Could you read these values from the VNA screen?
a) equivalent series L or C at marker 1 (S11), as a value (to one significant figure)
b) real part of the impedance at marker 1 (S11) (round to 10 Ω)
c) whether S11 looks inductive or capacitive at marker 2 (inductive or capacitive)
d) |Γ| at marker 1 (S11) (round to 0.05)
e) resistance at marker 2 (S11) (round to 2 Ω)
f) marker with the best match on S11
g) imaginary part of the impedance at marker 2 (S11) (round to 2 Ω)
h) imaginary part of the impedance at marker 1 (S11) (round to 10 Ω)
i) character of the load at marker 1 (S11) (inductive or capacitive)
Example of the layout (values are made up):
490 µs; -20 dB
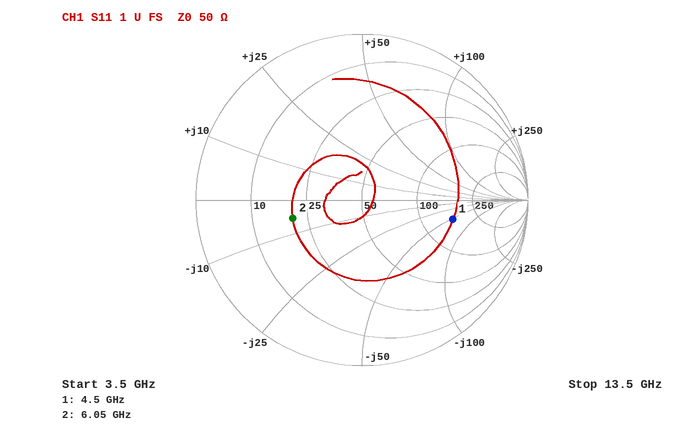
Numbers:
700 fF; 160 Ω; capacitive; 0.55; 20 Ω; marker 2; -6 Ω; -50 Ω; capacitive
